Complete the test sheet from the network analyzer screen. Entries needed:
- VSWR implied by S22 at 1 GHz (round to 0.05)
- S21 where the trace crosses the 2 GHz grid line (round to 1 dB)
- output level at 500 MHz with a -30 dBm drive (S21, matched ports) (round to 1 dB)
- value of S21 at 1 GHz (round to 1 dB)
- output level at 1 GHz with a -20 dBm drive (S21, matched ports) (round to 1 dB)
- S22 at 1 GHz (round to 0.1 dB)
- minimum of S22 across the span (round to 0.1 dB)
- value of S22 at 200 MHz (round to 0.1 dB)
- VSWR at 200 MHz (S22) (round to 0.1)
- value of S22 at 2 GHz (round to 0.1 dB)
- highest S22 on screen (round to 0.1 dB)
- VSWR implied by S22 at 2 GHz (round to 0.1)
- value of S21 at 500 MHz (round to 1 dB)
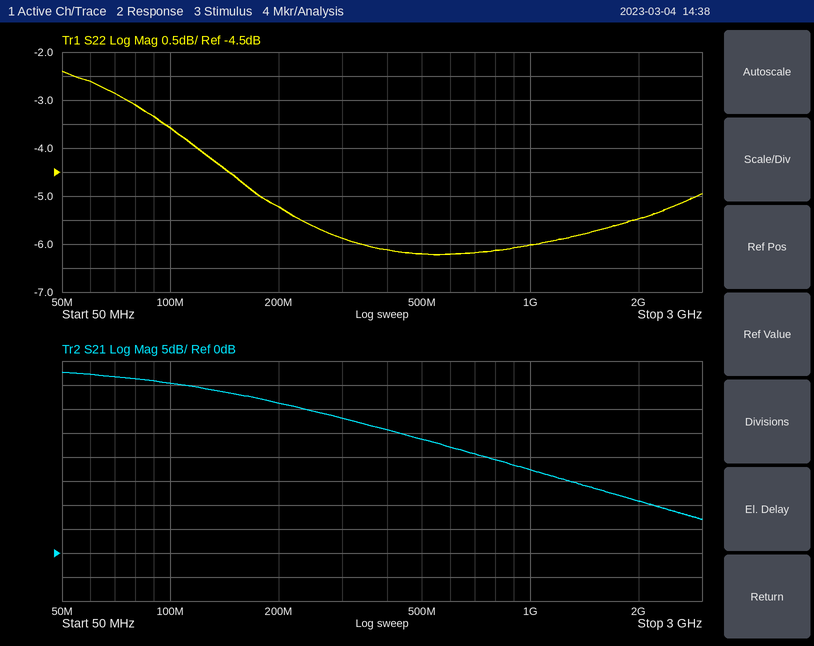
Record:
3.00
11 dB
-6 dBm
17 dB
-3 dBm
-6.0 dB
-6.2 dB
-5.2 dB
3.4
-5.5 dB
-2.4 dB
3.3
24 dB
